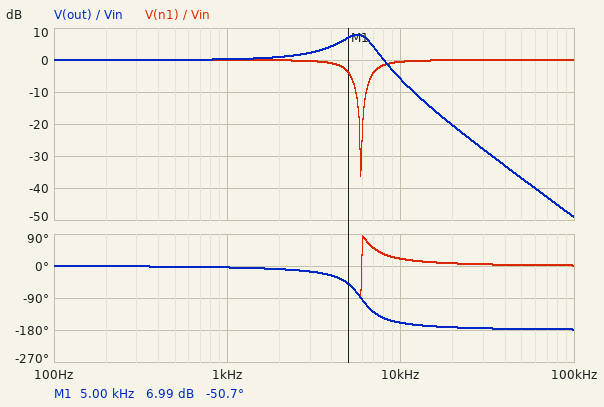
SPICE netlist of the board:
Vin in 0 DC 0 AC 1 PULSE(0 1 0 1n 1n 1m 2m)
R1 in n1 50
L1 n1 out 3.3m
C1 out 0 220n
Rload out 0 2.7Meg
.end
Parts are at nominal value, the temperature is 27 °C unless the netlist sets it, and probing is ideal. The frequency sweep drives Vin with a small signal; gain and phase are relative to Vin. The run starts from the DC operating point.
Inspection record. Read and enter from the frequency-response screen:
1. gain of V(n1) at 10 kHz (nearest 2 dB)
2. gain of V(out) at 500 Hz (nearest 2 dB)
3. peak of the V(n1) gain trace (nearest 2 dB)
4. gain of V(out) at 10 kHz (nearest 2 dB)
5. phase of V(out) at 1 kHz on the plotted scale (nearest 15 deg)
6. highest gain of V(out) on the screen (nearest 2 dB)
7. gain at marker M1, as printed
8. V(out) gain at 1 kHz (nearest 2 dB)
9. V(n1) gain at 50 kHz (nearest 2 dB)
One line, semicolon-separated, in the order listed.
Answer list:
0 dB; 0 dB; 0 dB; -6 dB; 0 deg; 8 dB; 6.99 dB; 0 dB; 0 dB
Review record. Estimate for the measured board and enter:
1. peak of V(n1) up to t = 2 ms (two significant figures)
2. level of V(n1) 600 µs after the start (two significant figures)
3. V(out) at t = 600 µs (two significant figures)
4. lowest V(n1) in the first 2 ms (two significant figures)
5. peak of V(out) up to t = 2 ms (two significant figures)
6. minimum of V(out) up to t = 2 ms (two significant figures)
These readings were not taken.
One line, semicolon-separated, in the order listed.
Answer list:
1.2 V; 1.0 V; 1.0 V; -160 mV; 1.5 V; -520 mV
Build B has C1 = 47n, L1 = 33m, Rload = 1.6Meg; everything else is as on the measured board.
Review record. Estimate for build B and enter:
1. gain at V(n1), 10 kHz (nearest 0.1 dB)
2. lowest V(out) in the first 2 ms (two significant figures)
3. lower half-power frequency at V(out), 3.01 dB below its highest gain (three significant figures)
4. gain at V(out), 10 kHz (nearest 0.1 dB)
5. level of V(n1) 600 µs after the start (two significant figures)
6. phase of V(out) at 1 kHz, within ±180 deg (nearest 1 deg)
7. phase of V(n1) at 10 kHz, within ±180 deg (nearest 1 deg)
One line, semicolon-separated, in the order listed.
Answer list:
0 dB; -510 mV; 3.91 kHz; -14.2 dB; 980 mV; -1 deg; 2 deg
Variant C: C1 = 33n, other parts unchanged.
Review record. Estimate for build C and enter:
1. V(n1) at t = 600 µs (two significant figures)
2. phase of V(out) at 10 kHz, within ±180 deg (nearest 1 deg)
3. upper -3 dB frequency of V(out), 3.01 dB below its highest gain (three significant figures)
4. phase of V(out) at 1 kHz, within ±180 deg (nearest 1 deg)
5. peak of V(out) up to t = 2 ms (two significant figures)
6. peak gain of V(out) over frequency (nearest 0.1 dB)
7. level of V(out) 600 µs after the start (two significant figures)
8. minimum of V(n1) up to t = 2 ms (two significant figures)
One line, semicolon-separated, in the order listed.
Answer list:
1.0 V; -10 deg; 16.3 kHz; -1 deg; 1.8 V; 16.0 dB; 990 mV; -110 mV
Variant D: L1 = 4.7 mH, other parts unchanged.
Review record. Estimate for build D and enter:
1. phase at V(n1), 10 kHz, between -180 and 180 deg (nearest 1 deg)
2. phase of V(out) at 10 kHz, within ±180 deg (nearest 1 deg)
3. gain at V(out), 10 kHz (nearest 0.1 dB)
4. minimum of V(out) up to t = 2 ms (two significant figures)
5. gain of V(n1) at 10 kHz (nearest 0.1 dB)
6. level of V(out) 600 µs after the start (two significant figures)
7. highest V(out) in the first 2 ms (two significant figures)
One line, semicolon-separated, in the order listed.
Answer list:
13 deg; -167 deg; -10.0 dB; -580 mV; -0.2 dB; 970 mV; 1.6 V
